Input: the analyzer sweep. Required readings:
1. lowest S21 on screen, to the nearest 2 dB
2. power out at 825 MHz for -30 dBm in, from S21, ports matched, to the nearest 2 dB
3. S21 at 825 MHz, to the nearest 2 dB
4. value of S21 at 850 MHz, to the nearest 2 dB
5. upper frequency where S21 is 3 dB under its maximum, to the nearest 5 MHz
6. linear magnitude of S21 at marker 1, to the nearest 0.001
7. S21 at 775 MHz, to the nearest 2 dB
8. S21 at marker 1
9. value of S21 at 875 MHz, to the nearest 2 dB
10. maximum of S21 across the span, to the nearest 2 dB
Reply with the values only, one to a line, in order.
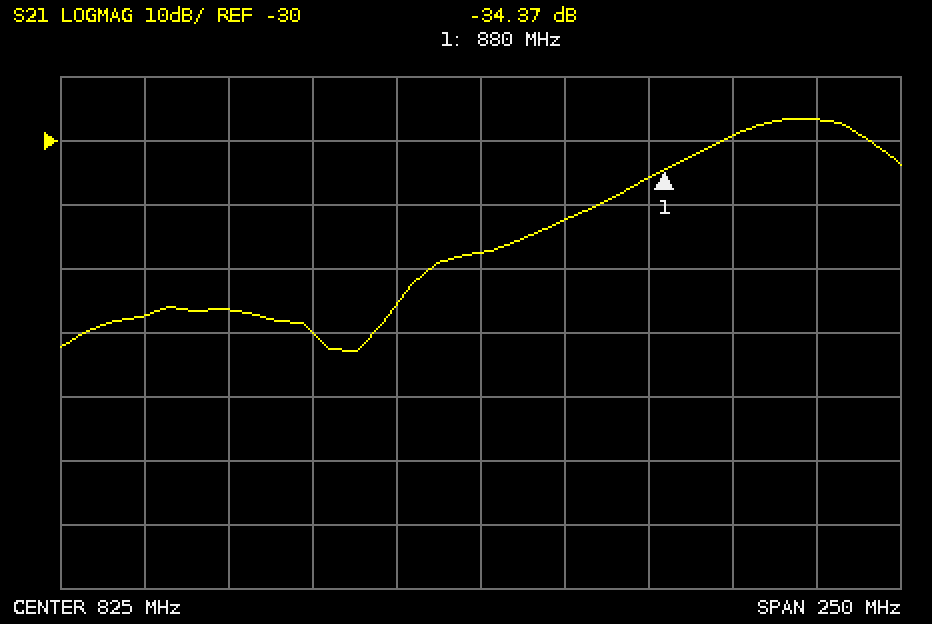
-62 dB
-78 dBm
-48 dB
-42 dB
940 MHz
0.019
-60 dB
-34.37 dB
-36 dB
-26 dB
